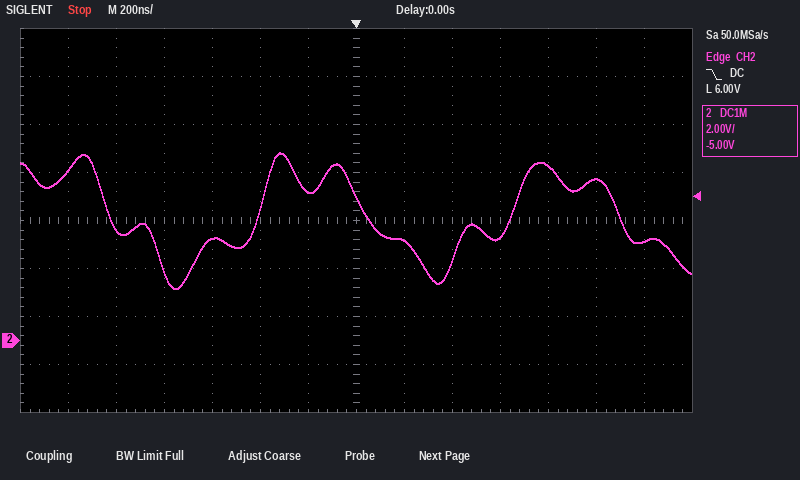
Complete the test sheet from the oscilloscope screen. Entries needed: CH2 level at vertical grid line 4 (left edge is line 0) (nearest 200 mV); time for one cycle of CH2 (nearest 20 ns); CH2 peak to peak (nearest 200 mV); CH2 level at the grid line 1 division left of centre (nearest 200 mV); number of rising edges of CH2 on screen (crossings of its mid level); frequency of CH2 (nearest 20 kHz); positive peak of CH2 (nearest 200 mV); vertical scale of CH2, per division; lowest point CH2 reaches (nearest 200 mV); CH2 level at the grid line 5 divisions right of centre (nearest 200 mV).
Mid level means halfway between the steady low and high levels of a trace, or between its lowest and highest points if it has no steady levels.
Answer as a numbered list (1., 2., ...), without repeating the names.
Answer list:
1. 4.2 V
2. 1.06 µs
3. 5.6 V
4. 6.2 V
5. 2
6. 940 kHz
7. 7.8 V
8. 2 V
9. 2.2 V
10. 6.8 V
